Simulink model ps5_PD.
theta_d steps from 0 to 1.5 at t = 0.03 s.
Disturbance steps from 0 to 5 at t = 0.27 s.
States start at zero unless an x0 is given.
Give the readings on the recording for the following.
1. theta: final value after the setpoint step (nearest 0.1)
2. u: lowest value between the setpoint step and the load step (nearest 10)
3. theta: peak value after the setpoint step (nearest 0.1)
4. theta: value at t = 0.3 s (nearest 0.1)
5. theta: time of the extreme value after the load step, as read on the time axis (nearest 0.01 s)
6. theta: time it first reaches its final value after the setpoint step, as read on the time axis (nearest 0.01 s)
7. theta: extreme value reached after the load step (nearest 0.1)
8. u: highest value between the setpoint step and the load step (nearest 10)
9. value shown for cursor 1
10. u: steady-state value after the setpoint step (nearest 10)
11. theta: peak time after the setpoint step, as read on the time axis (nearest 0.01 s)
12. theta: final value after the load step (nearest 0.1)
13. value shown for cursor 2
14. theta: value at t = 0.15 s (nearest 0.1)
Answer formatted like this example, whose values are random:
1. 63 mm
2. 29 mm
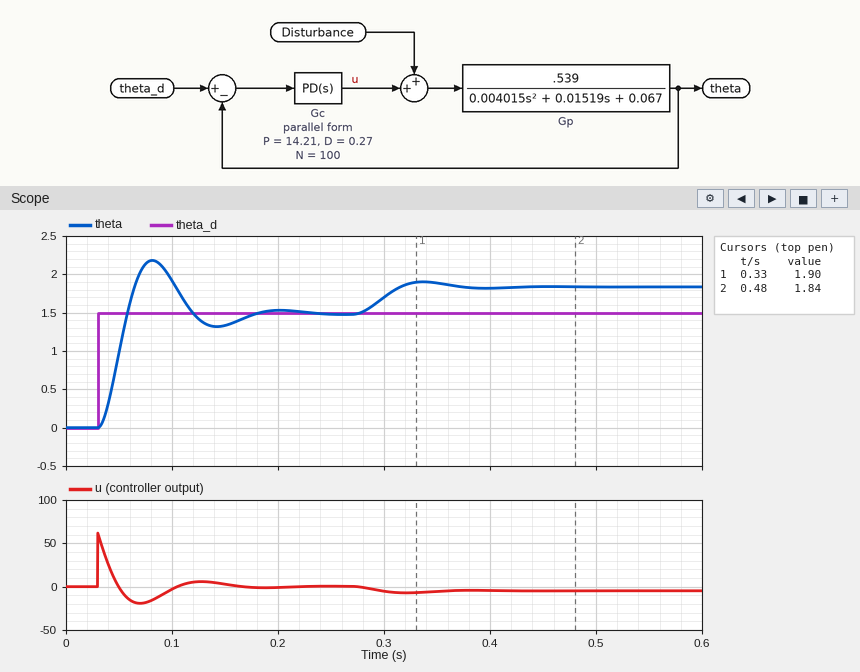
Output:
1. 1.5
2. -20
3. 2.2
4. 1.7
5. 0.34 s
6. 0.06 s
7. 1.9
8. 60
9. 1.90
10. 0
11. 0.08 s
12. 1.8
13. 1.84
14. 1.3
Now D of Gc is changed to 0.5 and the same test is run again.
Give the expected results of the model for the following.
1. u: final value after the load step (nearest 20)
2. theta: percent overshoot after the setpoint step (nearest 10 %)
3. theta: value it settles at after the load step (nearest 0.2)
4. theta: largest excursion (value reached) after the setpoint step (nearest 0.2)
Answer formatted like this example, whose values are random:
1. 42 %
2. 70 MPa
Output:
1. 0
2. 40 %
3. 1.8
4. 2.0
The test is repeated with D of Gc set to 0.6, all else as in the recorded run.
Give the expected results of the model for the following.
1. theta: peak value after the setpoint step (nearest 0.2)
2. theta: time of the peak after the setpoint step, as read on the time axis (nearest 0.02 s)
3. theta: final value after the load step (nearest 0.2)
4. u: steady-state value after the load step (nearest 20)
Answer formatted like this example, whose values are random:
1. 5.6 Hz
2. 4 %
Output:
1. 2.0
2. 0.06 s
3. 1.8
4. 0
